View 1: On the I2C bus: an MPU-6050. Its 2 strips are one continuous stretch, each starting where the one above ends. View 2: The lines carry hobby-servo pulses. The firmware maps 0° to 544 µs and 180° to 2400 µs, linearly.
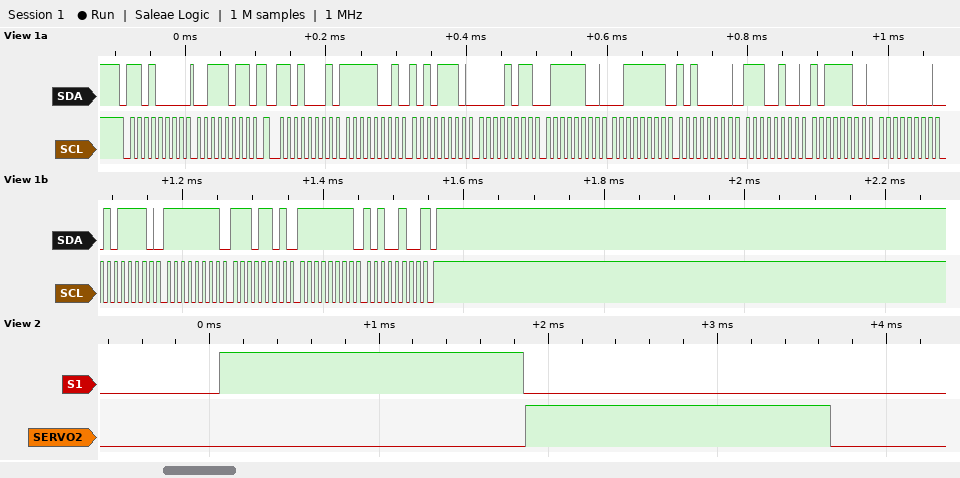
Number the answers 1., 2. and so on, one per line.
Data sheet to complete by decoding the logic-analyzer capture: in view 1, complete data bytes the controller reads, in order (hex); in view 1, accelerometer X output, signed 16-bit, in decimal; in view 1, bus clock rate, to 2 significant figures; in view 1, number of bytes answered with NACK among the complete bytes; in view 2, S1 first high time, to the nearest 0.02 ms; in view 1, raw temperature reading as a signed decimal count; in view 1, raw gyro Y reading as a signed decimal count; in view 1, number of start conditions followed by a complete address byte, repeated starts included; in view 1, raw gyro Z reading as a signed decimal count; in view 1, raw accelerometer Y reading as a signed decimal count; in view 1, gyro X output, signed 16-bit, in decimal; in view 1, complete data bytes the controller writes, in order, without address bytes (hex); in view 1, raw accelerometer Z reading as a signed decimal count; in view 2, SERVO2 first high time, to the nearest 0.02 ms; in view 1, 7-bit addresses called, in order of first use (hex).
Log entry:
1. F9 AE 0B 7C 3F A0 E4 BC 00 5E FF ED FF A4
2. -1618
3. 100 kHz
4. 1
5. 1.80 ms
6. -6980
7. -19
8. 2
9. -92
10. 2940
11. 94
12. 3B
13. 16288
14. 1.80 ms
15. 0x68
